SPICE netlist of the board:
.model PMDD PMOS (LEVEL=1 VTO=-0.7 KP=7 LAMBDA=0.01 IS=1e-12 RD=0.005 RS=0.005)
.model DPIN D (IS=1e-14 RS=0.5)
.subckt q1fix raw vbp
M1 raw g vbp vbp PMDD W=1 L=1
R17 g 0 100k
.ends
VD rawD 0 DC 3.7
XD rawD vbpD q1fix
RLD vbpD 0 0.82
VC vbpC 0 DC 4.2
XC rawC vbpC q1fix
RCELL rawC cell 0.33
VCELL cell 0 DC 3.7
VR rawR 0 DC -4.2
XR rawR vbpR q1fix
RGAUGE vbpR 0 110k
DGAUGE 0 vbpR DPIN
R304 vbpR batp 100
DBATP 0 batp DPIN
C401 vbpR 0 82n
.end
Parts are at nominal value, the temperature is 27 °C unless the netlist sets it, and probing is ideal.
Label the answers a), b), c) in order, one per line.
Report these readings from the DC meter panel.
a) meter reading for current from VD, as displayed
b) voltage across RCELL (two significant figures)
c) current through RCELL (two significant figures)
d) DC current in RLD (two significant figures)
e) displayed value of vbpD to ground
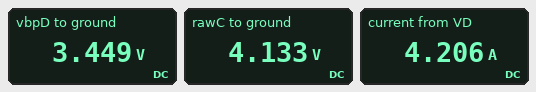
a) 4.206 A
b) 430 mV
c) 1.3 A
d) 4.2 A
e) 3.449 V
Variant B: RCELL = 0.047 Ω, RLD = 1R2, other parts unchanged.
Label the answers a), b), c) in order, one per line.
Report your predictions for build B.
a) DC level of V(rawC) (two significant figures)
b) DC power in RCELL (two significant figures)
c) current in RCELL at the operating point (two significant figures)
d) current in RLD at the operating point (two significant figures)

a) 3.9 V
b) 1.2 W
c) 5.0 A
d) 2.9 A
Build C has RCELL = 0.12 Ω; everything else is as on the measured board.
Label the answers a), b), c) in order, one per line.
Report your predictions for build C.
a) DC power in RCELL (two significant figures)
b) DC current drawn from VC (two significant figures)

a) 1.0 W
b) 2.9 A
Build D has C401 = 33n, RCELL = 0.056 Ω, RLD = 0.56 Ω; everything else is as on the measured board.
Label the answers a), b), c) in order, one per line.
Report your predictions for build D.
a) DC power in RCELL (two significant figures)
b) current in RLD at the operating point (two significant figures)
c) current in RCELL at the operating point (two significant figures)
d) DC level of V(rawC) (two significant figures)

a) 1.2 W
b) 6.0 A
c) 4.6 A
d) 4.0 V
